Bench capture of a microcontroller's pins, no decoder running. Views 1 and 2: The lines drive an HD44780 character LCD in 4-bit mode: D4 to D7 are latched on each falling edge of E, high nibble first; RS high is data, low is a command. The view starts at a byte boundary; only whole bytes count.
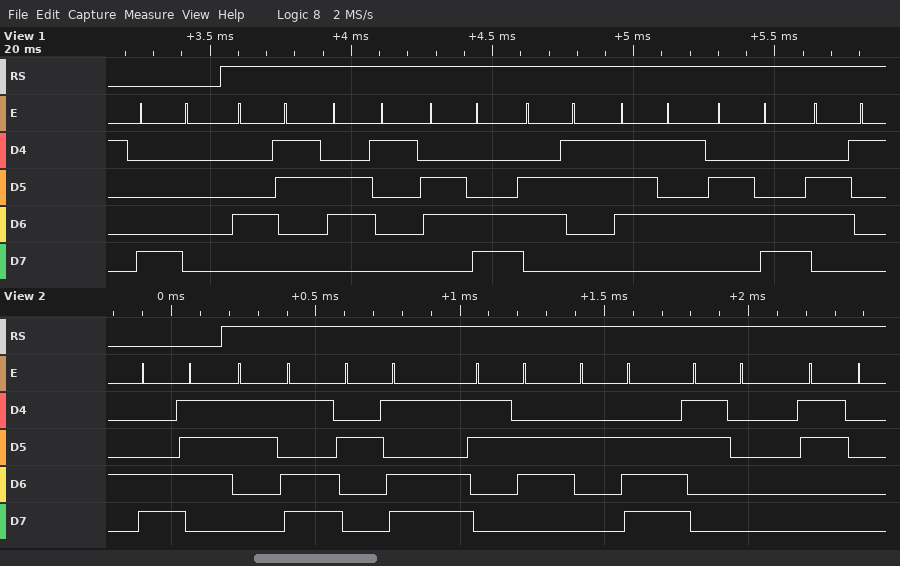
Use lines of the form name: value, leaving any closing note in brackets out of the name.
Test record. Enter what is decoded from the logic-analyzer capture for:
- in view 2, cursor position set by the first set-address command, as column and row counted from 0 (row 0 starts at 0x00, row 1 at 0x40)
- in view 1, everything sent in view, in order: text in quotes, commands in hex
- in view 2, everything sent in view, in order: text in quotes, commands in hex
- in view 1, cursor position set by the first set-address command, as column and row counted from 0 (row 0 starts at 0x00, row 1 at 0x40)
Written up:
in view 2, cursor position set by the first set-address command, as column and row counted from 0: column 7, row 1
in view 1, everything sent in view, in order: text in quotes, commands in hex: 0x80 "Calcula"
in view 2, everything sent in view, in order: text in quotes, commands in hex: 0xC7 "=-6.00"
in view 1, cursor position set by the first set-address command, as column and row counted from 0: column 0, row 0
